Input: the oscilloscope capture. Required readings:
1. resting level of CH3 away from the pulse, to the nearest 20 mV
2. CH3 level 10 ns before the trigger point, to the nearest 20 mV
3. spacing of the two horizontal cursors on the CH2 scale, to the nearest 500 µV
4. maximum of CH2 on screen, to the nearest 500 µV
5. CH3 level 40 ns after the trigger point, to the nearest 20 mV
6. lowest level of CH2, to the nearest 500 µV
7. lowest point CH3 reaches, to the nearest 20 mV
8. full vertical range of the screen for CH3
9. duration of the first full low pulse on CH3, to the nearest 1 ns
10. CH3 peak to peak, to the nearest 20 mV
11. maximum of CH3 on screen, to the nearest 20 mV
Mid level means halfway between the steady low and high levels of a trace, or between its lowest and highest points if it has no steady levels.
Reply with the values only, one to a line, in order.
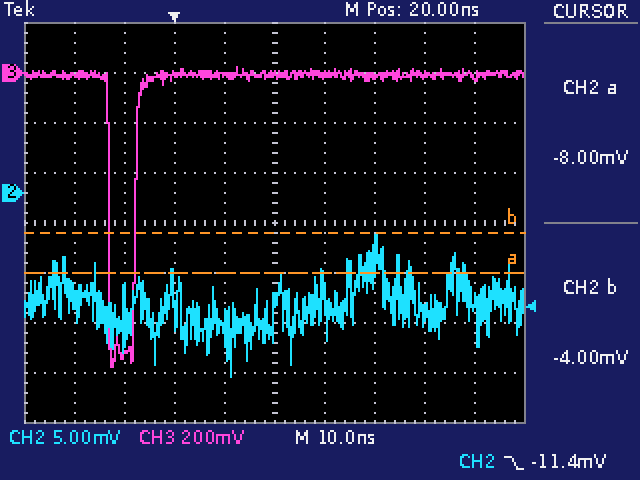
0 mV
-1.12 V
4.0 mV
-4.0 mV
-20 mV
-18.5 mV
-1.18 V
1.6 V
5 ns
1.20 V
20 mV
